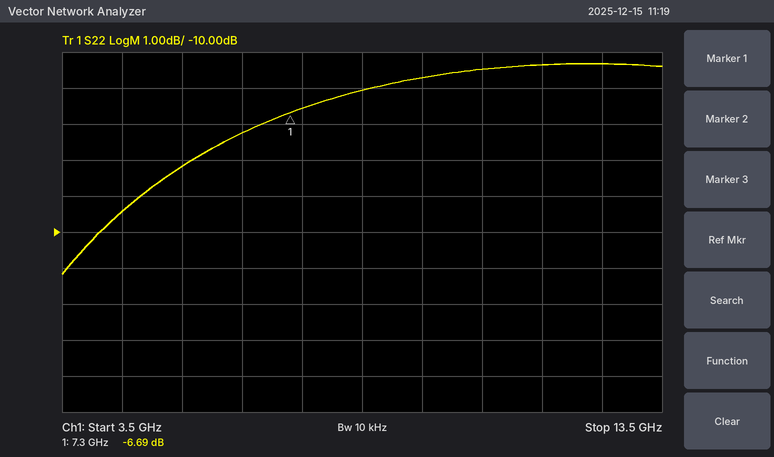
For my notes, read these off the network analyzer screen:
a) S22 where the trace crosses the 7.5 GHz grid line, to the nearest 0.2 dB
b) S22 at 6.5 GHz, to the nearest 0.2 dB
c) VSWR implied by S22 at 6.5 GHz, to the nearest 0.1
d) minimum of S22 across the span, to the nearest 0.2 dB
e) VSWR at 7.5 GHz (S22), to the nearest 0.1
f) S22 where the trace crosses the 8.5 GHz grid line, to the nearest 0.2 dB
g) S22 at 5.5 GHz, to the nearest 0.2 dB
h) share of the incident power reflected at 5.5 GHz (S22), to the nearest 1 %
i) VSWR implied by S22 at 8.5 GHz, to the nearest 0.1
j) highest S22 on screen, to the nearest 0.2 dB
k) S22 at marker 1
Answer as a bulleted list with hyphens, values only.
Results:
- -6.6 dB
- -7.2 dB
- 2.5
- -11.2 dB
- 2.8
- -6.0 dB
- -8.2 dB
- 15 %
- 3.0
- -5.4 dB
- -6.69 dB
